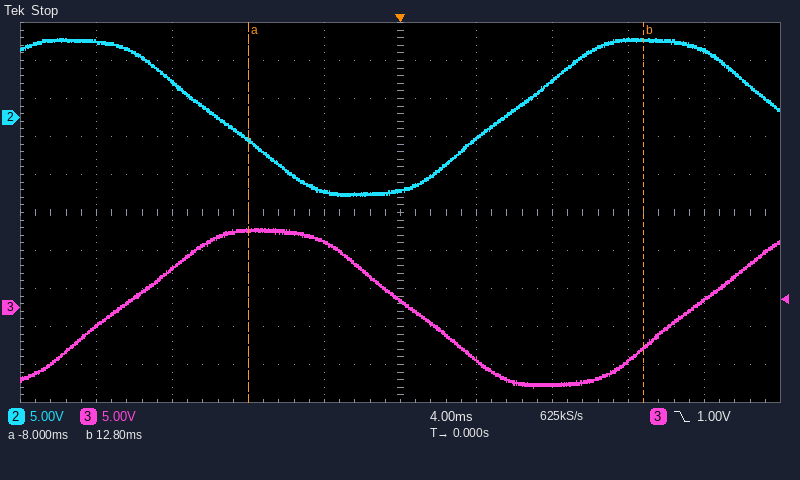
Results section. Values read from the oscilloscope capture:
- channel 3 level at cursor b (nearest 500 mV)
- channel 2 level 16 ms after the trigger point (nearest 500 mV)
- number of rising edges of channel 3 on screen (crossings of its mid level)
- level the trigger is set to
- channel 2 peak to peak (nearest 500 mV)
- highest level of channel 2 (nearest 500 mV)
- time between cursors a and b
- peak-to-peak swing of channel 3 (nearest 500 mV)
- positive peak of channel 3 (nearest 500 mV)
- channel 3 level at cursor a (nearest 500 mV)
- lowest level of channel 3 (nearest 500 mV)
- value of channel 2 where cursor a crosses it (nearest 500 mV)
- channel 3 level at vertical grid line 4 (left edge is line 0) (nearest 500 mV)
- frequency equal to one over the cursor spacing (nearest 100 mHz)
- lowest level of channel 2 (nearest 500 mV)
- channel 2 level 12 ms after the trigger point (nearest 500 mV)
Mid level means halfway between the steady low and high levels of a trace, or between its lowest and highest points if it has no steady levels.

-5.5 V
9.0 V
2
1.00 V
21.0 V
10.5 V
20.8 ms
21.0 V
10.5 V
10.0 V
-10.5 V
-3.0 V
8.5 V
48.1 Hz
-10.5 V
10.0 V
